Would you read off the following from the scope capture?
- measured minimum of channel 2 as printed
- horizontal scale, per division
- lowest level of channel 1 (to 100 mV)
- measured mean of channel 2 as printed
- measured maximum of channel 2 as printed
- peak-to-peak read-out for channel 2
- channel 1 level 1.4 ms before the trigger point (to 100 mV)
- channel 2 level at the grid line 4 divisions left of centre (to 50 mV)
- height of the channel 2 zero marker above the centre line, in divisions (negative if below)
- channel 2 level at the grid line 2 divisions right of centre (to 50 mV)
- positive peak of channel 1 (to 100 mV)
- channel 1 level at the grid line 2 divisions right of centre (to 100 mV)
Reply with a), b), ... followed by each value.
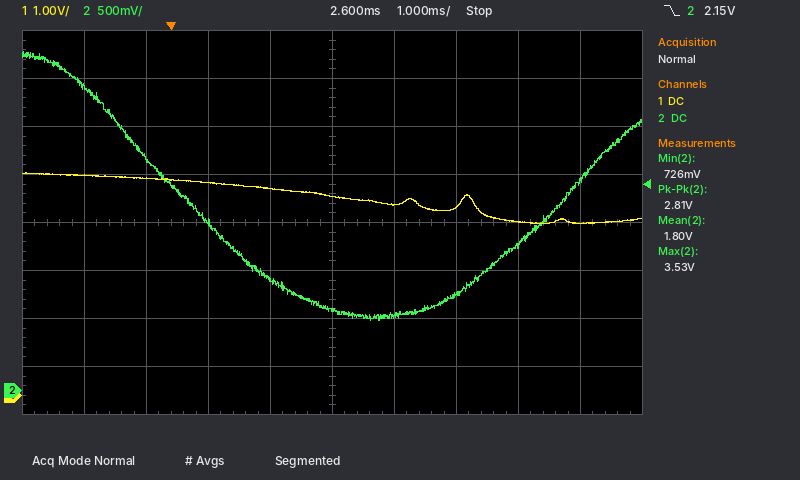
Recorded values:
a) 726 mV
b) 1 ms
c) 3.6 V
d) 1.80 V
e) 3.53 V
f) 2.81 V
g) 4.6 V
h) 3.15 V
i) -3.5 div
j) 1.00 V
k) 4.6 V
l) 3.9 V
